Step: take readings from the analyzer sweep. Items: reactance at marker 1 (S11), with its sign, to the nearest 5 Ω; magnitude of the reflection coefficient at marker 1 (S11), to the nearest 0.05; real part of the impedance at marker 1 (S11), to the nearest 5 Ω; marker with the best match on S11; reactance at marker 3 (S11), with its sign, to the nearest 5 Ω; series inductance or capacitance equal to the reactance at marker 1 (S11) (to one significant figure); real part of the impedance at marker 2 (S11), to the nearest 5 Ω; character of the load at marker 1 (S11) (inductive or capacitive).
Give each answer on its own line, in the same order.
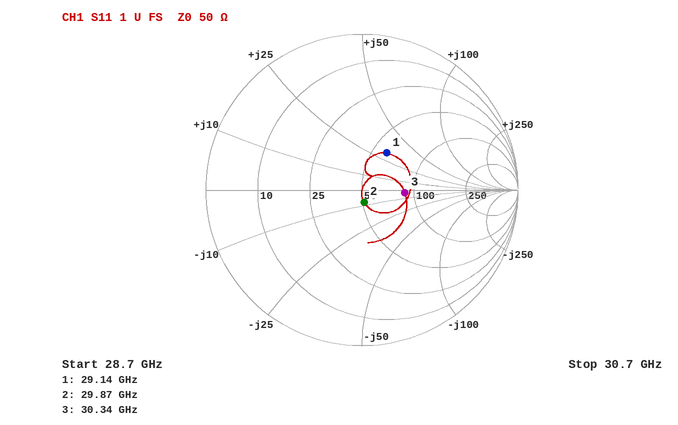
+30 Ω
0.30
60 Ω
marker 2
-5 Ω
200 pH
50 Ω
inductive
